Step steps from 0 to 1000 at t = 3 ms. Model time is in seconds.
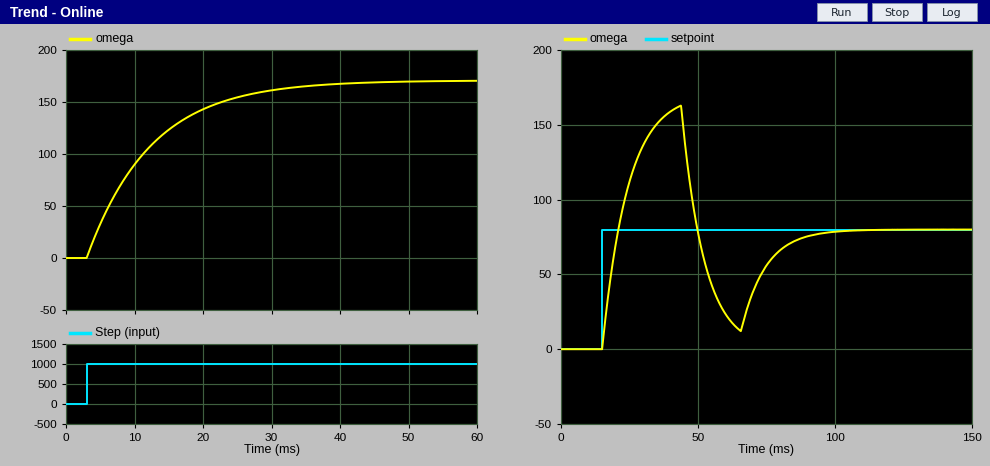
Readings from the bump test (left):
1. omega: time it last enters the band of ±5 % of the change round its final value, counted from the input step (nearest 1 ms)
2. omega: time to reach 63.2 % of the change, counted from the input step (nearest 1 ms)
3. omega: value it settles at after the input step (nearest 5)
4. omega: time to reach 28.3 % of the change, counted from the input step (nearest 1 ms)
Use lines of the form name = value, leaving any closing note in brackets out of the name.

omega: time it last enters the band of ±5 % of the change round its final value, counted from the input step = 28 ms
omega: time to reach 63.2 % of the change, counted from the input step = 9 ms
omega: value it settles at after the input step = 170
omega: time to reach 28.3 % of the change, counted from the input step = 3 ms
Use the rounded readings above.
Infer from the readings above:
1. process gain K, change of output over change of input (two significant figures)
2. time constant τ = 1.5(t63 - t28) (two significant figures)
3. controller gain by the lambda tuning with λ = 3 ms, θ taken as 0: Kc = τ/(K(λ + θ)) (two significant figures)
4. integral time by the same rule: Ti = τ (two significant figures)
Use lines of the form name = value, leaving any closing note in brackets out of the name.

process gain K, change of output over change of input = 0.17
time constant τ = 1.5(t63 - t28) = 9.0 ms
controller gain by the lambda tuning with λ = 3 ms, θ taken as 0: Kc = τ/(K(λ + θ)) = 18
integral time by the same rule: Ti = τ = 9.0 ms
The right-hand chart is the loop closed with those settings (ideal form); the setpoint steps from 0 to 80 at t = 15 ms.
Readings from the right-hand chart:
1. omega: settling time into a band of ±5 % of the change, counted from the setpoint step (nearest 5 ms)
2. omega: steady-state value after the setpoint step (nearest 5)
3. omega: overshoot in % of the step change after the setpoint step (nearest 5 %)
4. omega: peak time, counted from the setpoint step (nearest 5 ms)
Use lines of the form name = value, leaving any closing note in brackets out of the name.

omega: settling time into a band of ±5 % of the change, counted from the setpoint step = 75 ms
omega: steady-state value after the setpoint step = 80
omega: overshoot in % of the step change after the setpoint step = 105 %
omega: peak time, counted from the setpoint step = 30 ms
